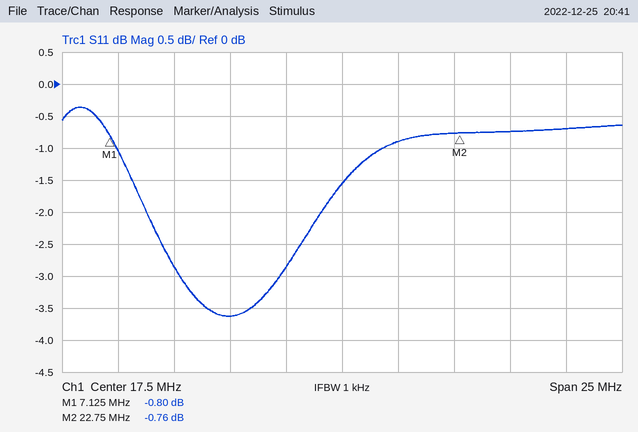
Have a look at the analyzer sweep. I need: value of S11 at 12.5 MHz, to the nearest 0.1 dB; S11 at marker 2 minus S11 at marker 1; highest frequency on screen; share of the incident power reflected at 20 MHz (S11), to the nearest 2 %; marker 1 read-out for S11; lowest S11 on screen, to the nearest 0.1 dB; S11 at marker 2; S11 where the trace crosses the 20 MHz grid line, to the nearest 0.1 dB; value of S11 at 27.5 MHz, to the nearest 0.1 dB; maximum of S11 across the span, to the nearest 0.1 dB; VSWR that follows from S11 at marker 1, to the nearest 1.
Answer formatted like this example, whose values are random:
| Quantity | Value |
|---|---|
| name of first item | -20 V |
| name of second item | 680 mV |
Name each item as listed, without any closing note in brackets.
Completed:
| Quantity | Value |
|---|---|
| value of S11 at 12.5 MHz, to the nearest 0.1 dB | -3.6 dB |
| S11 at marker 2 minus S11 at marker 1 | 0.04 dB |
| highest frequency on screen | 30 MHz |
| share of the incident power reflected at 20 MHz (S11), to the nearest 2 % | 82 % |
| marker 1 read-out for S11 | -0.80 dB |
| lowest S11 on screen, to the nearest 0.1 dB | -3.6 dB |
| S11 at marker 2 | -0.76 dB |
| S11 where the trace crosses the 20 MHz grid line, to the nearest 0.1 dB | -0.9 dB |
| value of S11 at 27.5 MHz, to the nearest 0.1 dB | -0.7 dB |
| maximum of S11 across the span, to the nearest 0.1 dB | -0.4 dB |
| VSWR that follows from S11 at marker 1, to the nearest 1 | 22 |
